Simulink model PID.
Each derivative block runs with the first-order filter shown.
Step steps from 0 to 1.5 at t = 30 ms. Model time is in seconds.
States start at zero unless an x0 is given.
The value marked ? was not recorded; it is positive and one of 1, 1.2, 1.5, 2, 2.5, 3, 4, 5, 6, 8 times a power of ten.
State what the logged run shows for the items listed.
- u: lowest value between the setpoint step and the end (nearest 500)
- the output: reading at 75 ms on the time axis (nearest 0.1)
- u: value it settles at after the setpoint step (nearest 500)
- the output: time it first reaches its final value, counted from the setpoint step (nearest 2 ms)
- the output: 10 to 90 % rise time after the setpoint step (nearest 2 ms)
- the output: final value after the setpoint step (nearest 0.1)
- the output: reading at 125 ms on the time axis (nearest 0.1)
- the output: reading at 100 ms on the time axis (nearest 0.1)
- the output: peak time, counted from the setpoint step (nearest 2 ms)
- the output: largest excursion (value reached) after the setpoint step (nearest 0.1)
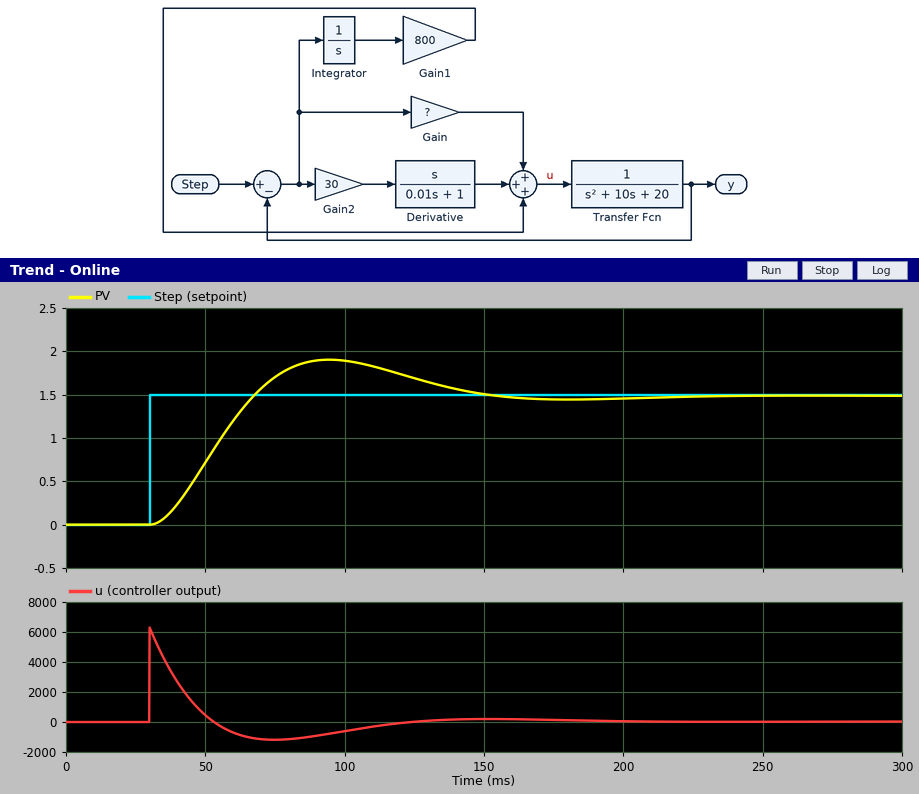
-1000
1.7
0
38 ms
26 ms
1.5
1.7
1.9
64 ms
1.9
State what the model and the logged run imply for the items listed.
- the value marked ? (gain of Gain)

1200
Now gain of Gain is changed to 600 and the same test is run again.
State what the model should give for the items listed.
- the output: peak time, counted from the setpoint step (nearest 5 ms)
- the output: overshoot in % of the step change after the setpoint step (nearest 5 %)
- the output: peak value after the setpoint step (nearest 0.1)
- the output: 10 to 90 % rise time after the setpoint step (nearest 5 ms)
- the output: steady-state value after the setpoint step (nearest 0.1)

80 ms
10 %
1.7
35 ms
1.5
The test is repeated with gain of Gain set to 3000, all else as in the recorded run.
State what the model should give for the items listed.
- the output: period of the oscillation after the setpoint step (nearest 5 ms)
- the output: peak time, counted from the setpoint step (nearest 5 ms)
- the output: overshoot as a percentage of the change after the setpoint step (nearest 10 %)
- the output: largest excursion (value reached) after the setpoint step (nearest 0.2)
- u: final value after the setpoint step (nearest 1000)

100 ms
45 ms
50 %
2.2
0
